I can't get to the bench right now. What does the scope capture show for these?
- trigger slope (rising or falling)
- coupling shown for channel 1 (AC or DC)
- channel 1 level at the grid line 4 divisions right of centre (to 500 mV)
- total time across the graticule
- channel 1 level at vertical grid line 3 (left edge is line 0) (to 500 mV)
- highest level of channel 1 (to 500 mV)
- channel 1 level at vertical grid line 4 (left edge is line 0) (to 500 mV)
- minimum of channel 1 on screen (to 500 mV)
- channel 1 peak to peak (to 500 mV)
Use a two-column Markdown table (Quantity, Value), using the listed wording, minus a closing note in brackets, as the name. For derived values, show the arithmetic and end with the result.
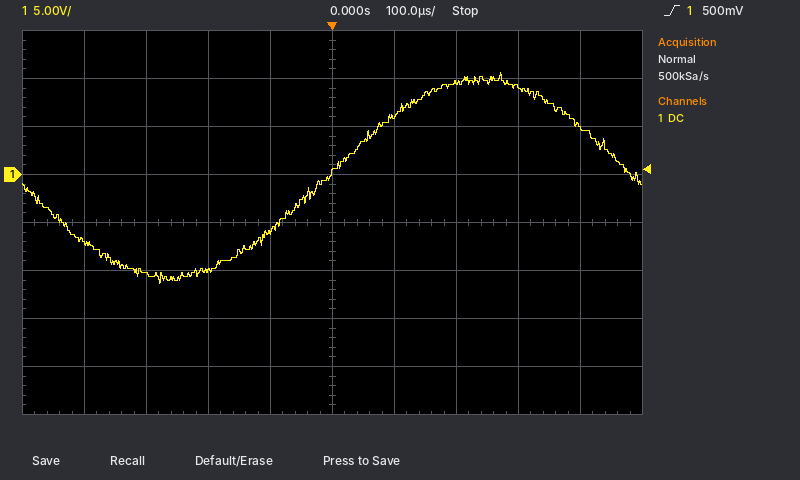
| Quantity | Value |
|---|---|
| trigger slope | rising |
| coupling shown for channel 1 | DC |
| channel 1 level at the grid line 4 divisions right of centre | 5.0 V |
| total time across the graticule | 1 ms |
| channel 1 level at vertical grid line 3 (left edge is line 0) | -10.0 V |
| highest level of channel 1 | 10.5 V |
| channel 1 level at vertical grid line 4 (left edge is line 0) | -6.0 V |
| minimum of channel 1 on screen | -11.5 V |
| channel 1 peak to peak | 10.5 V − (-11.5 V) = 22.0 V |
